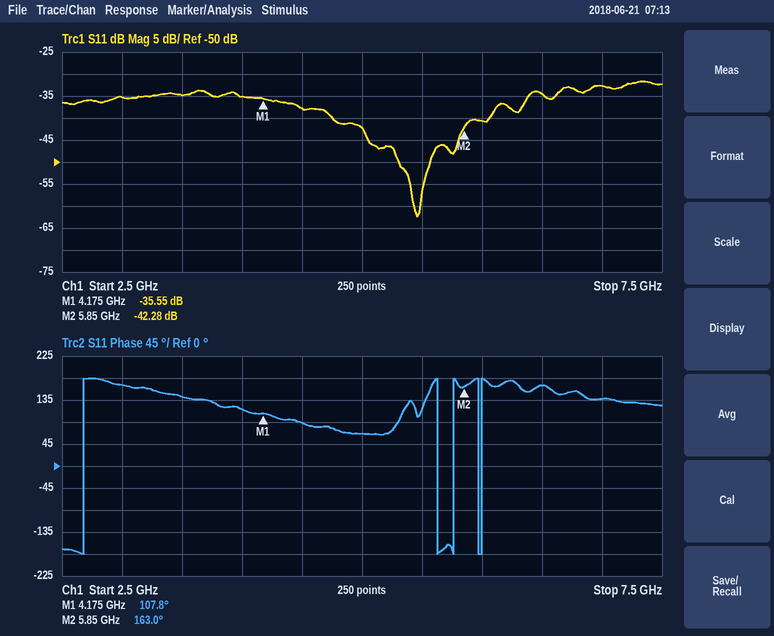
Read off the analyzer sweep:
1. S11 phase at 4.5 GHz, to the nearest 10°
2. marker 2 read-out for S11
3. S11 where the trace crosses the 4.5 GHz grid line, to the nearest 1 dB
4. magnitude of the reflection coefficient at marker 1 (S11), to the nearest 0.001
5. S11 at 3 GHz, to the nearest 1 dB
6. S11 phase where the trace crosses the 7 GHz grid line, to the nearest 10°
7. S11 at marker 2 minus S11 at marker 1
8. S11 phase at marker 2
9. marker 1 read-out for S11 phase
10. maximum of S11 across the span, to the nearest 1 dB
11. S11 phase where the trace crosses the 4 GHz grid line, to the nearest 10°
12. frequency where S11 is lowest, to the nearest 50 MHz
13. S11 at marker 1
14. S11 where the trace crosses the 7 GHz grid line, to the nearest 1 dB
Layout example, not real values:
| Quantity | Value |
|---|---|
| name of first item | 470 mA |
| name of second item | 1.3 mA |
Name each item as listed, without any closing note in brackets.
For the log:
| Quantity | Value |
|---|---|
| S11 phase at 4.5 GHz, to the nearest 10° | 90° |
| marker 2 read-out for S11 | -42.28 dB |
| S11 where the trace crosses the 4.5 GHz grid line, to the nearest 1 dB | -38 dB |
| magnitude of the reflection coefficient at marker 1 (S11), to the nearest 0.001 | 0.017 |
| S11 at 3 GHz, to the nearest 1 dB | -35 dB |
| S11 phase where the trace crosses the 7 GHz grid line, to the nearest 10° | 140° |
| S11 at marker 2 minus S11 at marker 1 | -6.73 dB |
| S11 phase at marker 2 | 163.0° |
| marker 1 read-out for S11 phase | 107.8° |
| maximum of S11 across the span, to the nearest 1 dB | -32 dB |
| S11 phase where the trace crosses the 4 GHz grid line, to the nearest 10° | 120° |
| frequency where S11 is lowest, to the nearest 50 MHz | 5.45 GHz |
| S11 at marker 1 | -35.55 dB |
| S11 where the trace crosses the 7 GHz grid line, to the nearest 1 dB | -33 dB |
